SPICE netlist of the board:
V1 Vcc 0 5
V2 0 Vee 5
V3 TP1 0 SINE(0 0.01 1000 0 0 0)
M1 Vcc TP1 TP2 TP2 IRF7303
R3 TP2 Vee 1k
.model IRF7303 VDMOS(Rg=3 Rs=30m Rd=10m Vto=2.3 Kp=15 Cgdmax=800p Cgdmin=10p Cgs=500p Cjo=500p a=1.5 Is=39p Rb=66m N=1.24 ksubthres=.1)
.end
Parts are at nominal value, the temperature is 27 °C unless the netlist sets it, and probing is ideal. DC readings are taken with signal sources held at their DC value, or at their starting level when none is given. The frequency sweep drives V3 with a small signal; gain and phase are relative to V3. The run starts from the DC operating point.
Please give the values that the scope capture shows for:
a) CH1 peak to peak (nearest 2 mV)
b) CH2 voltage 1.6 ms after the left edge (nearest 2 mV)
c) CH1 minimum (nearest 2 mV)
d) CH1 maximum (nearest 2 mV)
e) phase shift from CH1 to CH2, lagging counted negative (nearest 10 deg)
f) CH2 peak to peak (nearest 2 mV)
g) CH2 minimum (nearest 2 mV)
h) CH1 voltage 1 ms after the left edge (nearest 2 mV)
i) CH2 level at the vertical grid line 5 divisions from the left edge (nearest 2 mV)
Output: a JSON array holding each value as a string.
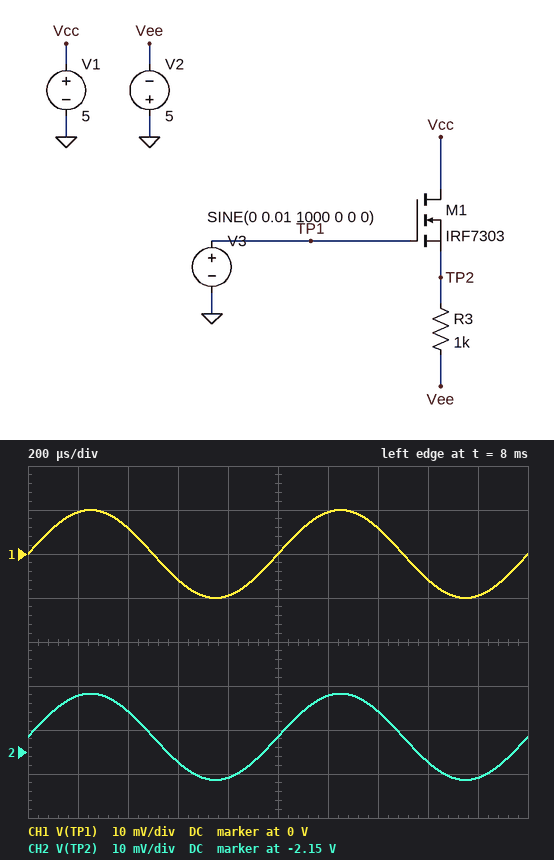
["20 mV", "-2.152 V", "-10 mV", "10 mV", "0 deg", "20 mV", "-2.156 V", "0 V", "-2.146 V"]
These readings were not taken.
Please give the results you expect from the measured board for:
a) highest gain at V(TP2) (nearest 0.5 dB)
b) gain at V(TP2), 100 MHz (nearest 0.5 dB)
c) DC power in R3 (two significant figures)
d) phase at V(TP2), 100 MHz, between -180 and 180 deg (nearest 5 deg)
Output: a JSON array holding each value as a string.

["0 dB", "-2.5 dB", "8.1 mW", "-20 deg"]
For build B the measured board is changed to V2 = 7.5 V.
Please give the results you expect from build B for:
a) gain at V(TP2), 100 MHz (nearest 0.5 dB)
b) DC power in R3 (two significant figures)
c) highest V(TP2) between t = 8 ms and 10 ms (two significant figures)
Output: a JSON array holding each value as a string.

["-2.5 dB", "28 mW", "-2.2 V"]
